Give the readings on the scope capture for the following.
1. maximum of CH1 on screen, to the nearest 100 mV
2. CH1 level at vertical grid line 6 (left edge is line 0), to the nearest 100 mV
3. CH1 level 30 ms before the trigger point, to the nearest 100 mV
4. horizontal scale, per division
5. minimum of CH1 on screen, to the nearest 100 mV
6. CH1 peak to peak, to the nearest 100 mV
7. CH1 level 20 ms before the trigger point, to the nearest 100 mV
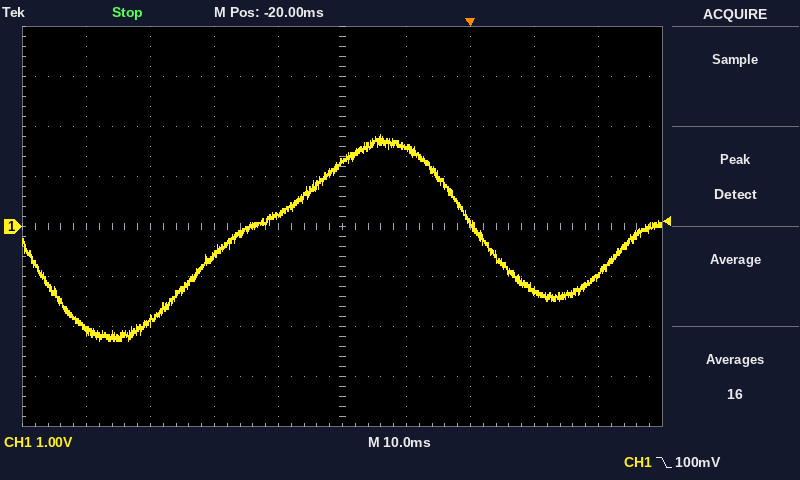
1.8 V
1.6 V
200 mV
10 ms
-2.3 V
4.1 V
1.3 V
